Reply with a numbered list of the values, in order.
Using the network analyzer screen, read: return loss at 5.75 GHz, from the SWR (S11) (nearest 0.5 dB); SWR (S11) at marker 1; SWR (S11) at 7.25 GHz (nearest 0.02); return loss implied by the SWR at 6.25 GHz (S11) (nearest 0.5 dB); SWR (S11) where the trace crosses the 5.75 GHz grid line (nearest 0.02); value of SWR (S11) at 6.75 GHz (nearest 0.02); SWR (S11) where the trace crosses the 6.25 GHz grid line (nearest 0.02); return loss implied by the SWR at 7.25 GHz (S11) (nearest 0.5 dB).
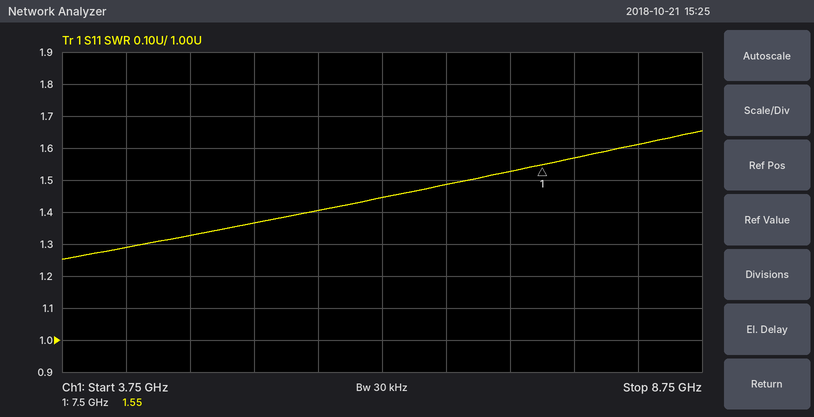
1. 15.5 dB
2. 1.55
3. 1.52
4. 15.0 dB
5. 1.40
6. 1.48
7. 1.44
8. 13.5 dB
